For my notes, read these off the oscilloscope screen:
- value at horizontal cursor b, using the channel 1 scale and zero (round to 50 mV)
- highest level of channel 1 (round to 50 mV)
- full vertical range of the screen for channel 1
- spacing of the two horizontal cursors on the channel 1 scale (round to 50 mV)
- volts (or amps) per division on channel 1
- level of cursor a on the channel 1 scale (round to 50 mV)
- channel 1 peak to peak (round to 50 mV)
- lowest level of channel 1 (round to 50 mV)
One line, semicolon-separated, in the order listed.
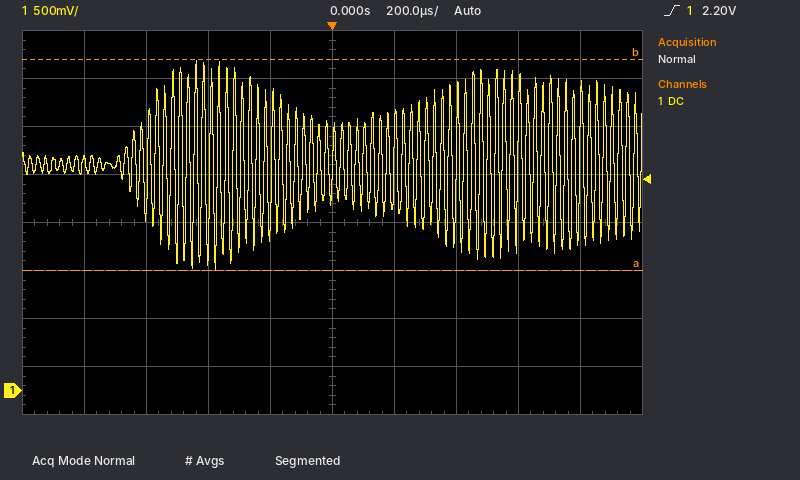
3.45 V; 3.45 V; 4 V; 2.20 V; 500 mV; 1.25 V; 2.20 V; 1.25 V
